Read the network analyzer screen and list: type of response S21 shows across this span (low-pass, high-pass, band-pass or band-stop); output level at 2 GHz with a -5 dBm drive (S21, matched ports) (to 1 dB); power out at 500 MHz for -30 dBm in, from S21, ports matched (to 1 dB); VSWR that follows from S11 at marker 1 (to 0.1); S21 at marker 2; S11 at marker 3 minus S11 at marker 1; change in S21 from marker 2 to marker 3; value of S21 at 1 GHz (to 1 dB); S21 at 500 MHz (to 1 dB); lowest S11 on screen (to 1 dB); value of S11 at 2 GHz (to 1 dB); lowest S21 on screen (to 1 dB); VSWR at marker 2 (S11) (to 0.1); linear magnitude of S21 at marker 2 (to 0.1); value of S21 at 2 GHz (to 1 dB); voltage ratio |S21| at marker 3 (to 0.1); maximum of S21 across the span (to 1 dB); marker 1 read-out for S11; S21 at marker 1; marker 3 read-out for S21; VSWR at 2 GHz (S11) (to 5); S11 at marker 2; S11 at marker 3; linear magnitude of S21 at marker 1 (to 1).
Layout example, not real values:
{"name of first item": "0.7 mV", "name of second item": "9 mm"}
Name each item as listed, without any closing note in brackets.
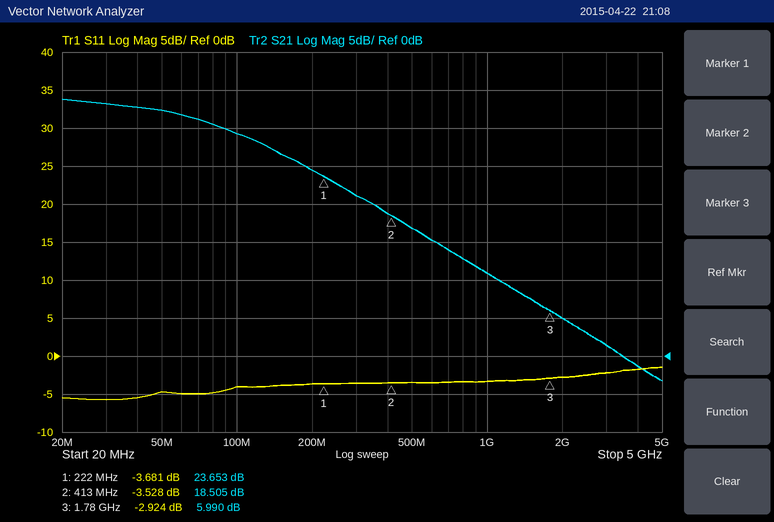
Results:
{"type of response S21 shows across this span": "low-pass", "output level at 2 GHz with a -5 dBm drive (S21, matched ports)": "0 dBm", "power out at 500 MHz for -30 dBm in, from S21, ports matched": "-13 dBm", "VSWR that follows from S11 at marker 1": "4.8", "S21 at marker 2": "18.505 dB", "S11 at marker 3 minus S11 at marker 1": "0.757 dB", "change in S21 from marker 2 to marker 3": "-12.515 dB", "value of S21 at 1 GHz": "11 dB", "S21 at 500 MHz": "17 dB", "lowest S11 on screen": "-6 dB", "value of S11 at 2 GHz": "-3 dB", "lowest S21 on screen": "-3 dB", "VSWR at marker 2 (S11)": "5.0", "linear magnitude of S21 at marker 2": "8.4", "value of S21 at 2 GHz": "5 dB", "voltage ratio |S21| at marker 3": "2.0", "maximum of S21 across the span": "34 dB", "marker 1 read-out for S11": "-3.681 dB", "S21 at marker 1": "23.653 dB", "marker 3 read-out for S21": "5.990 dB", "VSWR at 2 GHz (S11)": "5", "S11 at marker 2": "-3.528 dB", "S11 at marker 3": "-2.924 dB", "linear magnitude of S21 at marker 1": "15"}
